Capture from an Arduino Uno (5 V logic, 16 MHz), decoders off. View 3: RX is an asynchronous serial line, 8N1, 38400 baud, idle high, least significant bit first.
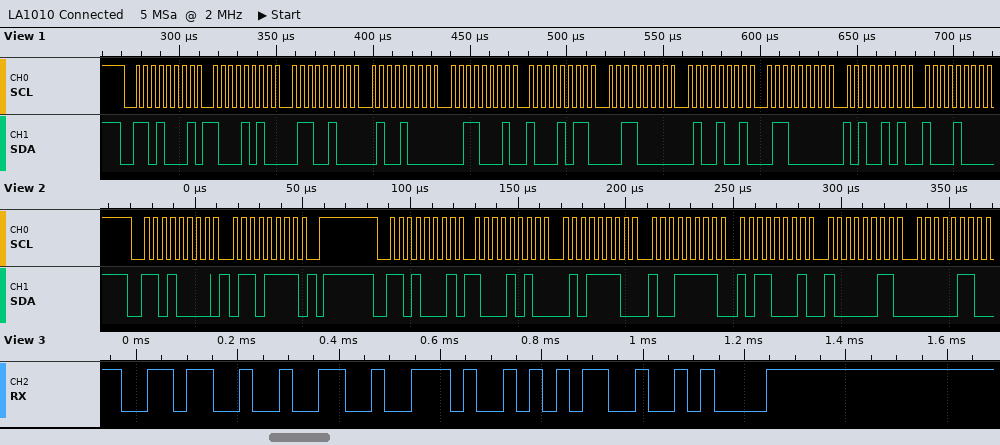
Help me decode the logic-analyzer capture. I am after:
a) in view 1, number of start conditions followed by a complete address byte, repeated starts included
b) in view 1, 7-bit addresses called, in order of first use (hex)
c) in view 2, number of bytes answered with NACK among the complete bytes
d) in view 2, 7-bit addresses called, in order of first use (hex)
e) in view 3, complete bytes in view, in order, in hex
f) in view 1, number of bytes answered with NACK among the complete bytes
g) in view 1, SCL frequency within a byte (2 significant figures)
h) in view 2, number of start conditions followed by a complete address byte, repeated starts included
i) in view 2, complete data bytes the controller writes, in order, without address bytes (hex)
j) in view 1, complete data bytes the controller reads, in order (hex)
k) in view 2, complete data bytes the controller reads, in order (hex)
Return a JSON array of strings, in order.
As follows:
["1", "0x68", "0", "0x68", "36 32 2E 35 0A", "0", "250 kHz", "2", "6F", "8A 64 48 31 8B 30 49 60 A5 88", "8A 5E 9F B1 83 06"]
